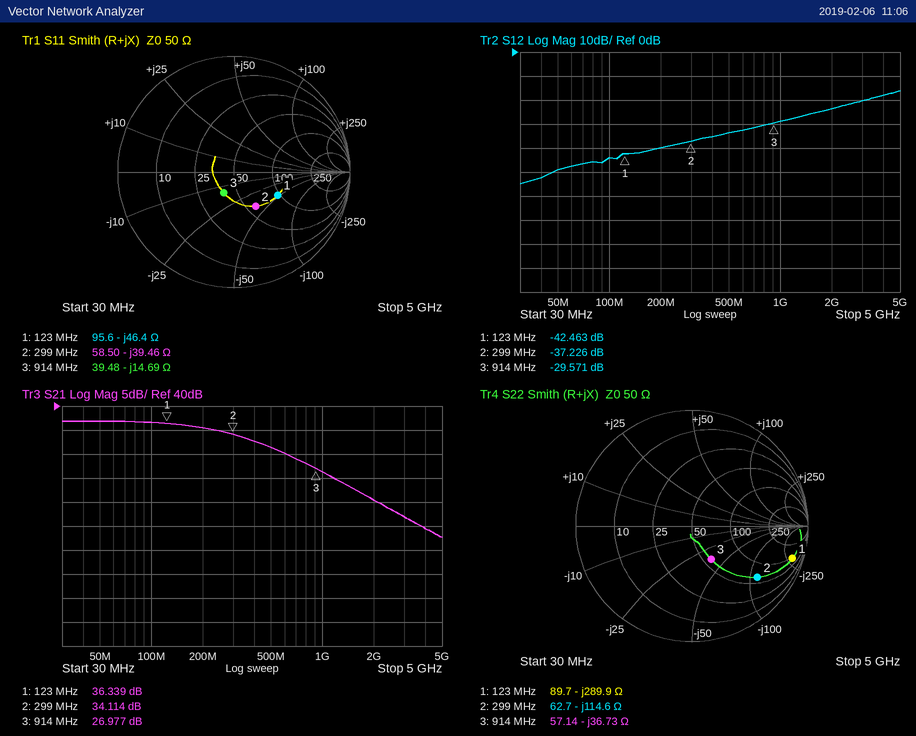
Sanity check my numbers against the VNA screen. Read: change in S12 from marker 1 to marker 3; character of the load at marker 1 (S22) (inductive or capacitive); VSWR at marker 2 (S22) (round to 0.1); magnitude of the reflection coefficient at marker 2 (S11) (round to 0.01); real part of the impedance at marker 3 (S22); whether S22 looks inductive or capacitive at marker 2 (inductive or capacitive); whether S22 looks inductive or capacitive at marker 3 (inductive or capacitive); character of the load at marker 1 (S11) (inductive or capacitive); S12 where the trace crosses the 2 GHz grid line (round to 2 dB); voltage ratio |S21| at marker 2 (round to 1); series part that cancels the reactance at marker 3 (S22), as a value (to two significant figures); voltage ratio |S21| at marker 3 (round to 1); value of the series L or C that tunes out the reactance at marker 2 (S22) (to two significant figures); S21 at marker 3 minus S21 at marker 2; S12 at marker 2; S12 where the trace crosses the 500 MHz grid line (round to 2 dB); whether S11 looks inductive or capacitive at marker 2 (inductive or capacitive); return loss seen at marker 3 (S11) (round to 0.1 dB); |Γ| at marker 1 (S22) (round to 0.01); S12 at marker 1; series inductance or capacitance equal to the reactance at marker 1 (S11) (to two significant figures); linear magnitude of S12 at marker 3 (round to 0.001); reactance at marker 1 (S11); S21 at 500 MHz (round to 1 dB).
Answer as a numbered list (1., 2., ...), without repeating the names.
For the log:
1. 12.892 dB
2. capacitive
3. 6.1
4. 0.35
5. 57.14 Ω
6. capacitive
7. capacitive
8. capacitive
9. -24 dB
10. 51
11. 6.4 nH
12. 22
13. 61 nH
14. -7.137 dB
15. -37.226 dB
16. -34 dB
17. capacitive
18. 14.0 dB
19. 0.91
20. -42.463 dB
21. 28 pF
22. 0.033
23. -46.4 Ω
24. 31 dB
